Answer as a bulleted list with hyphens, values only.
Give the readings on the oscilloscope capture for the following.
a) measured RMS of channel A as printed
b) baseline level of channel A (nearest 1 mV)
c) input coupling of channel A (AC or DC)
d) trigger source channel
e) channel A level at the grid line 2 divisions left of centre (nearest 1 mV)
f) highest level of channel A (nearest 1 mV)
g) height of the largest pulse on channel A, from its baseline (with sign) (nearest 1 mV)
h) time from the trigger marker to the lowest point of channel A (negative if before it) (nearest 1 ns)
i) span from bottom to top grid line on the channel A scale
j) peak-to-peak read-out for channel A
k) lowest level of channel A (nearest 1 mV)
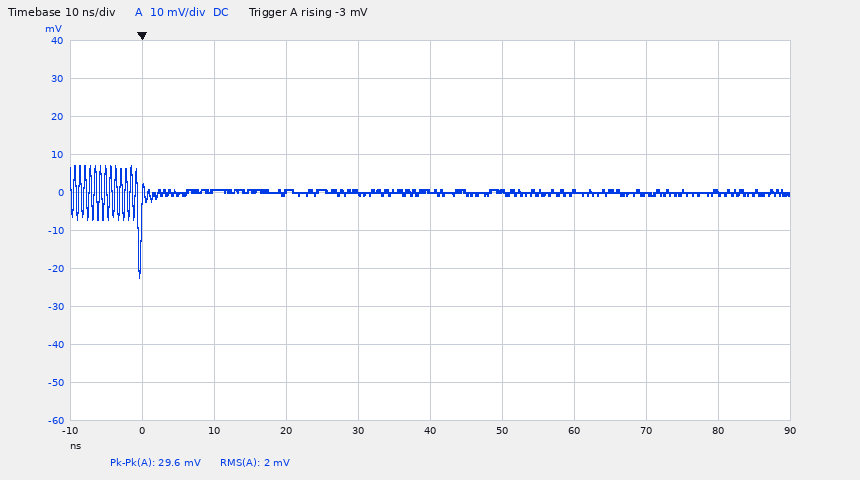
- 2 mV
- 0 mV
- DC
- channel A
- 0 mV
- 7 mV
- -22 mV
- 0 ns
- 100 mV
- 29.6 mV
- -22 mV
